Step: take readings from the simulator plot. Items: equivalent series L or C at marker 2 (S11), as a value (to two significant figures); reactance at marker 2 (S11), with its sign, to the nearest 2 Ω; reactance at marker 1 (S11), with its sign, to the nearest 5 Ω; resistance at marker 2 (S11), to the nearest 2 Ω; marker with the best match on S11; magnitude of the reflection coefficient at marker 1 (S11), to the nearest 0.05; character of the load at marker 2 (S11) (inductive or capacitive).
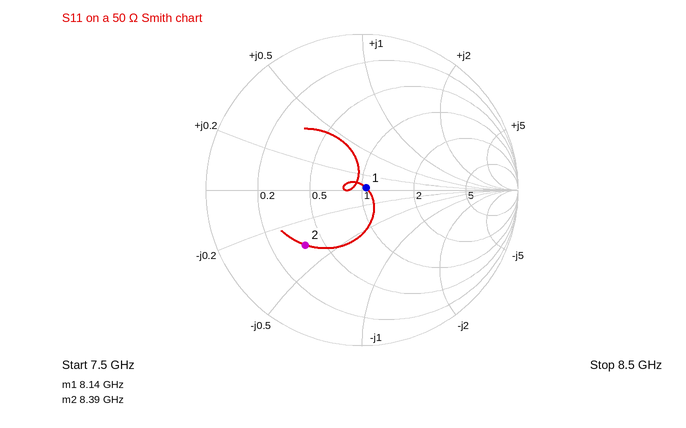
1.1 pF
-18 Ω
0 Ω
18 Ω
marker 1
0.05
capacitive
